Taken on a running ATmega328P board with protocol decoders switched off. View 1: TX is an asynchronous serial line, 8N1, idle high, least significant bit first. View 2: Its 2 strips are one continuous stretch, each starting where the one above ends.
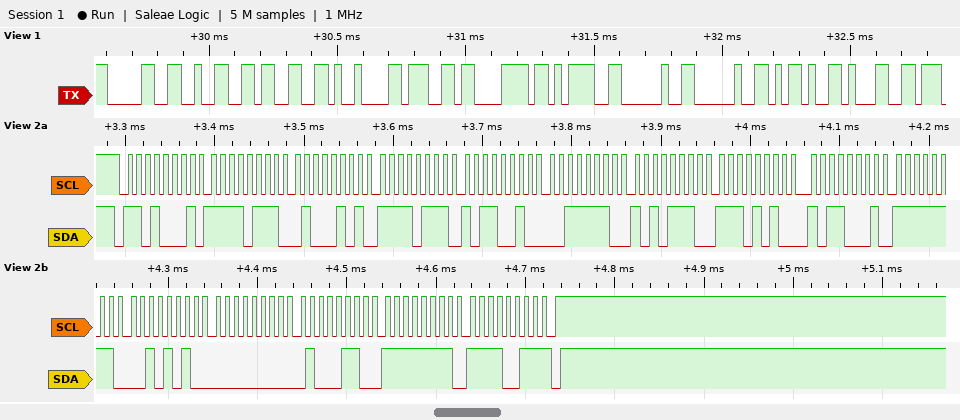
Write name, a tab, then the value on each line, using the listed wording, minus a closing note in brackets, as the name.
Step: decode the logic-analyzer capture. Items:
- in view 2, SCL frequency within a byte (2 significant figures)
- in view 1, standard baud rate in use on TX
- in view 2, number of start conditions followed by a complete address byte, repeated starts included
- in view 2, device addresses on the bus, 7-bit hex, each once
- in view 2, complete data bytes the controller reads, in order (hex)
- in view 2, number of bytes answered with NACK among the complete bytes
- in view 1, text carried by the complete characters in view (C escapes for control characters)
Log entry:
in view 2, SCL frequency within a byte	100 kHz
in view 1, standard baud rate in use on TX	38400 baud
in view 2, number of start conditions followed by a complete address byte, repeated starts included	1
in view 2, device addresses on the bus, 7-bit hex, each once	0x68
in view 2, complete data bytes the controller reads, in order	F7 45 F7 B2 3E AE EA B1 FF 2A 00 46 FF F3
in view 2, number of bytes answered with NACK among the complete bytes	1
in view 1, text carried by the complete characters in view	"023\tgx=  -1"
